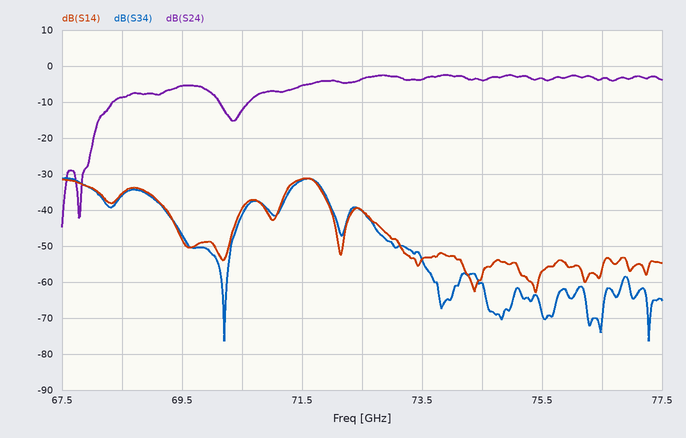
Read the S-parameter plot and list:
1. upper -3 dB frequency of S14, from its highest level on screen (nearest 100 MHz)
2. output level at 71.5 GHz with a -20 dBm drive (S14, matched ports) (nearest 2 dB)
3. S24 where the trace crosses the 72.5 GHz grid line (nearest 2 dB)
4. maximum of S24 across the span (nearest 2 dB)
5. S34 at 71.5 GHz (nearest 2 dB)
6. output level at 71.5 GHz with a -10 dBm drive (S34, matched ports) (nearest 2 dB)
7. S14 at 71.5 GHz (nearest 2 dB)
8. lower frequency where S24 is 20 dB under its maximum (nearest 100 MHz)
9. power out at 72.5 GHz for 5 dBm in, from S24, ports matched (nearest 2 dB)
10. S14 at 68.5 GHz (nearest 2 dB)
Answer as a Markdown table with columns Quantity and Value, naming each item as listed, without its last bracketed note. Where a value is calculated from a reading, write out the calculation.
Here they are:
| Quantity | Value |
|---|---|
| upper -3 dB frequency of S14, from its highest level on screen | 71.8 GHz |
| output level at 71.5 GHz with a -20 dBm drive (S14, matched ports) | -20 dBm + (-32 dB) = -52 dBm |
| S24 where the trace crosses the 72.5 GHz grid line | -4 dB |
| maximum of S24 across the span | -2 dB |
| S34 at 71.5 GHz | -32 dB |
| output level at 71.5 GHz with a -10 dBm drive (S34, matched ports) | -10 dBm + (-32 dB) = -42 dBm |
| S14 at 71.5 GHz | -32 dB |
| lower frequency where S24 is 20 dB under its maximum | 68.0 GHz |
| power out at 72.5 GHz for 5 dBm in, from S24, ports matched | 5 dBm + (-4 dB) = 2 dBm |
| S14 at 68.5 GHz | -36 dB |
